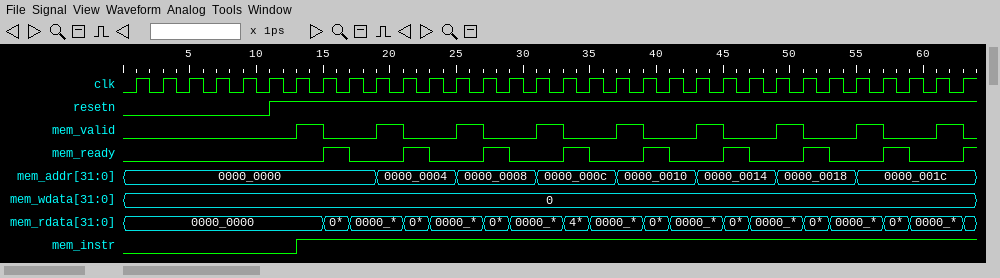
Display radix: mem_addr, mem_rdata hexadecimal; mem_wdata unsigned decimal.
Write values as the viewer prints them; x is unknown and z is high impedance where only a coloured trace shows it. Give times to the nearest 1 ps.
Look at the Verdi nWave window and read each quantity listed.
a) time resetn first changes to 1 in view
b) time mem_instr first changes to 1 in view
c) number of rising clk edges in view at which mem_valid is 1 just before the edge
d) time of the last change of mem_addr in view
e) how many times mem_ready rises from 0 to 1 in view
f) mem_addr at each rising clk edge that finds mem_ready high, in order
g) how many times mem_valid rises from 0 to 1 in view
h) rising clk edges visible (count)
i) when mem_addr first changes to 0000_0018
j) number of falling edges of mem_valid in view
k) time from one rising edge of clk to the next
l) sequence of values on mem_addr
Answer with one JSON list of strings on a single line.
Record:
["11 ps", "13 ps", "9", "55 ps", "9", "0000_0000, 0000_0004, 0000_0008, 0000_000c, 0000_0010, 0000_0014, 0000_0018, 0000_001c", "9", "32", "49 ps", "9", "2 ps", "0000_0000, 0000_0004, 0000_0008, 0000_000c, 0000_0010, 0000_0014, 0000_0018, 0000_001c"]
